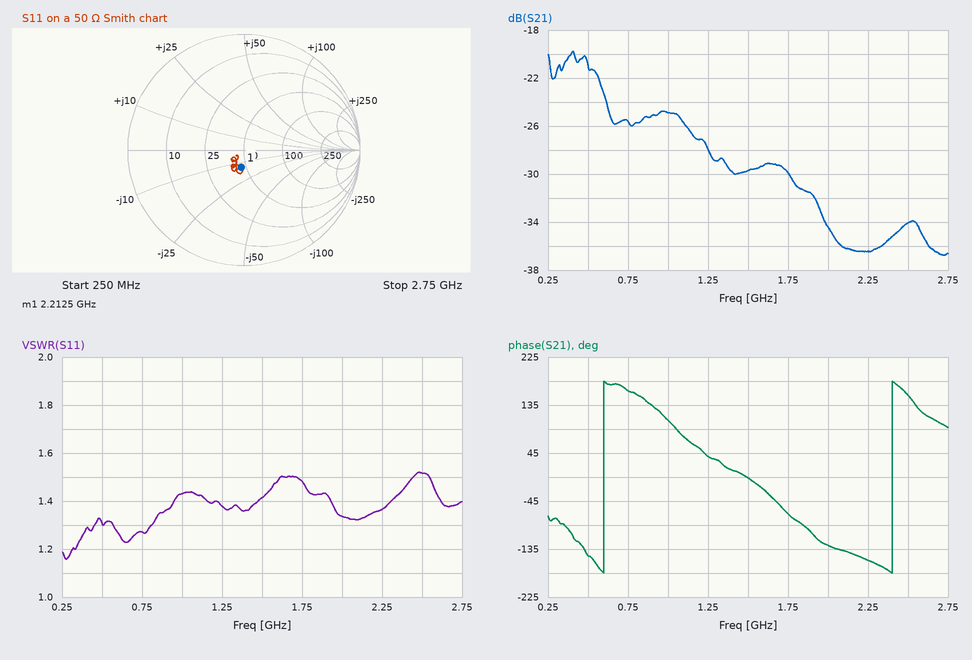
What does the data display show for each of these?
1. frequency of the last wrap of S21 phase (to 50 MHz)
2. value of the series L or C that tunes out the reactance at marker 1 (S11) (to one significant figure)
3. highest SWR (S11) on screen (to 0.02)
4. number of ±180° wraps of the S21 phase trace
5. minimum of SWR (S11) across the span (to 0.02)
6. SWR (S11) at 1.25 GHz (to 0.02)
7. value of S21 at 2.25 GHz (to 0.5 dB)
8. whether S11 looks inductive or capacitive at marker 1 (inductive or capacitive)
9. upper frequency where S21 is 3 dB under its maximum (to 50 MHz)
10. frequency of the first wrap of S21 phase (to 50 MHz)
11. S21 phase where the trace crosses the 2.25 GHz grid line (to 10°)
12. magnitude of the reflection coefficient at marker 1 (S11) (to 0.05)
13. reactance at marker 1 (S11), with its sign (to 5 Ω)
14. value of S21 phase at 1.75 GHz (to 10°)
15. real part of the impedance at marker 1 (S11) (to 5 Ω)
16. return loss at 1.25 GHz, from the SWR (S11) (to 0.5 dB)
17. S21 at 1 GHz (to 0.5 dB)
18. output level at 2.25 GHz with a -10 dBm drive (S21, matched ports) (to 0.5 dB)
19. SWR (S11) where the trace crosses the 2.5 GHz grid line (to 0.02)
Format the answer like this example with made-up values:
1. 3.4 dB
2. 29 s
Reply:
1. 2.40 GHz
2. 1 nH
3. 1.52
4. 2
5. 1.16
6. 1.38
7. -36.5 dB
8. capacitive
9. 600 MHz
10. 600 MHz
11. -160°
12. 0.15
13. -15 Ω
14. -70°
15. 45 Ω
16. 16.0 dB
17. -25.0 dB
18. -46.5 dBm
19. 1.52
